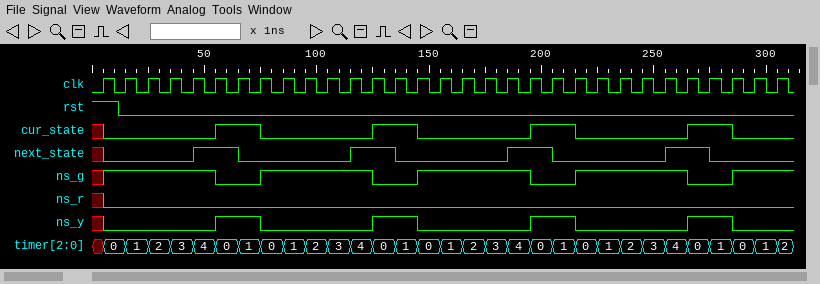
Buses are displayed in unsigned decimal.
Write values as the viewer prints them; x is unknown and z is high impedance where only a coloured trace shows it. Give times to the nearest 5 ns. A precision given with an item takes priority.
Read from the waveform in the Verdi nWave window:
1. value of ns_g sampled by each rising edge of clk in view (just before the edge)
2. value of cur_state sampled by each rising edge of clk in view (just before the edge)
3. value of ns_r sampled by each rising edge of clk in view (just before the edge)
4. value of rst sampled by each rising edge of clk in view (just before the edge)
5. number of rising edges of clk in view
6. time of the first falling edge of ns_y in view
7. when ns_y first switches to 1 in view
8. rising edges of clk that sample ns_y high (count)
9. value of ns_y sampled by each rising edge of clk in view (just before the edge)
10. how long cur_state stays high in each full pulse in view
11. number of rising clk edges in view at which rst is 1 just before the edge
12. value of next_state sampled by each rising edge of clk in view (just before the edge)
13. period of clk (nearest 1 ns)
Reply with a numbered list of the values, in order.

1. x 1 1 1 1 1 0 0 1 1 1 1 1 0 0 1 1 1 1 1 0 0 1 1 1 1 1 0 0 1 1
2. x 0 0 0 0 0 1 1 0 0 0 0 0 1 1 0 0 0 0 0 1 1 0 0 0 0 0 1 1 0 0
3. x 0 0 0 0 0 0 0 0 0 0 0 0 0 0 0 0 0 0 0 0 0 0 0 0 0 0 0 0 0 0
4. 1 0 0 0 0 0 0 0 0 0 0 0 0 0 0 0 0 0 0 0 0 0 0 0 0 0 0 0 0 0 0
5. 31
6. 75 ns
7. 55 ns
8. 8
9. x 0 0 0 0 0 1 1 0 0 0 0 0 1 1 0 0 0 0 0 1 1 0 0 0 0 0 1 1 0 0
10. 20 ns, 20 ns, 20 ns, 20 ns
11. 1
12. x 0 0 0 0 1 1 0 0 0 0 0 1 1 0 0 0 0 0 1 1 0 0 0 0 0 1 1 0 0 0
13. 10 ns
